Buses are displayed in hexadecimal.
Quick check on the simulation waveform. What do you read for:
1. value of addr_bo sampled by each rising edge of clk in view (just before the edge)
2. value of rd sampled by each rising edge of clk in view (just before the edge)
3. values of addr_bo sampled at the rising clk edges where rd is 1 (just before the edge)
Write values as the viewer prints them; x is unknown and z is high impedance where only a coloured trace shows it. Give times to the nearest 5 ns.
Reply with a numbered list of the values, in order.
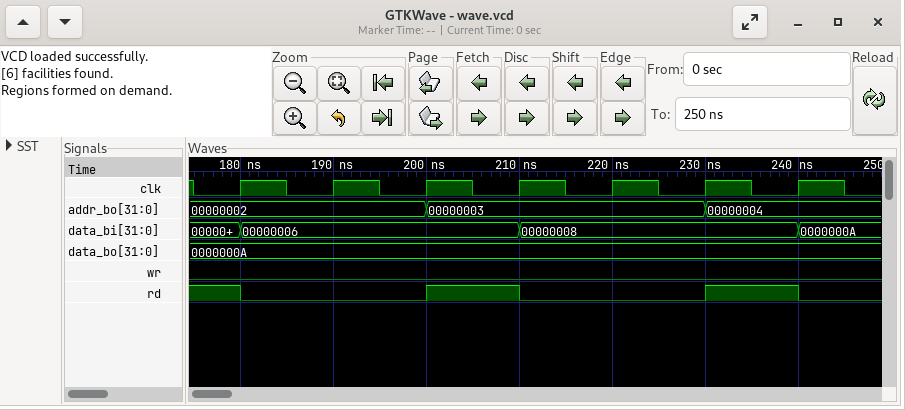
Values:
1. 00000002, 00000002, 00000002, 00000003, 00000003, 00000003, 00000004
2. 1 0 0 1 0 0 1
3. 00000002, 00000003, 00000004
